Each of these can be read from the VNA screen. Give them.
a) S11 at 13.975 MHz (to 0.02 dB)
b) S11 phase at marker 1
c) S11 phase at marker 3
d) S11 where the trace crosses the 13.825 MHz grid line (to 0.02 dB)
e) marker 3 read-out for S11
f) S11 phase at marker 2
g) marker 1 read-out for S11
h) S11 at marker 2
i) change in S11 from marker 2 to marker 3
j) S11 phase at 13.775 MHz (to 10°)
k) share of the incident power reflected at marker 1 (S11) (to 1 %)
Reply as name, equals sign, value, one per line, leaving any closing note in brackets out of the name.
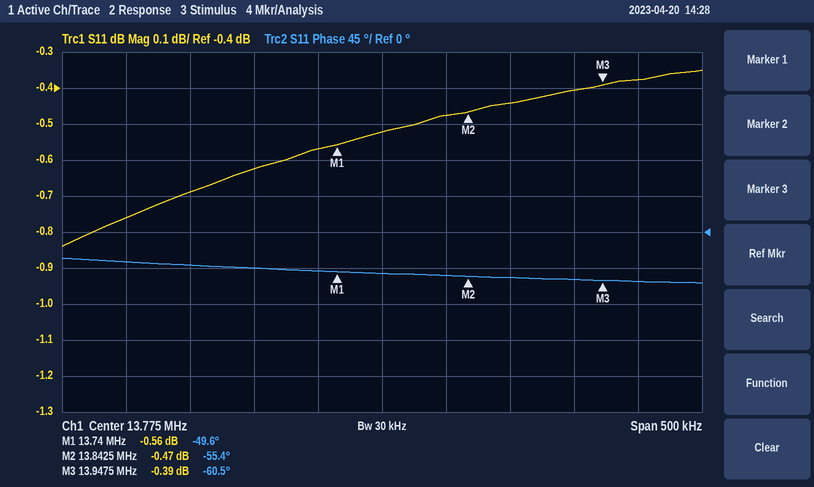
S11 at 13.975 MHz = -0.38 dB
S11 phase at marker 1 = -49.6°
S11 phase at marker 3 = -60.5°
S11 where the trace crosses the 13.825 MHz grid line = -0.48 dB
marker 3 read-out for S11 = -0.39 dB
S11 phase at marker 2 = -55.4°
marker 1 read-out for S11 = -0.56 dB
S11 at marker 2 = -0.47 dB
change in S11 from marker 2 to marker 3 = 0.08 dB
S11 phase at 13.775 MHz = -50°
share of the incident power reflected at marker 1 (S11) = 88 %
